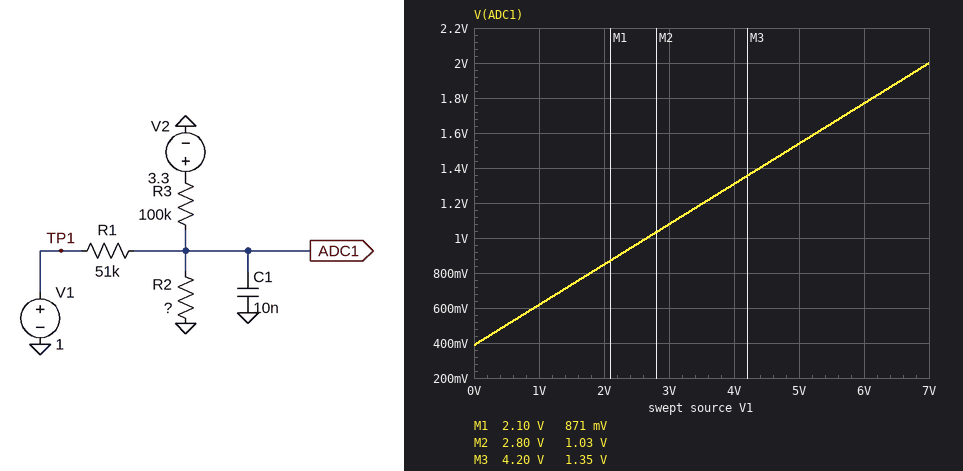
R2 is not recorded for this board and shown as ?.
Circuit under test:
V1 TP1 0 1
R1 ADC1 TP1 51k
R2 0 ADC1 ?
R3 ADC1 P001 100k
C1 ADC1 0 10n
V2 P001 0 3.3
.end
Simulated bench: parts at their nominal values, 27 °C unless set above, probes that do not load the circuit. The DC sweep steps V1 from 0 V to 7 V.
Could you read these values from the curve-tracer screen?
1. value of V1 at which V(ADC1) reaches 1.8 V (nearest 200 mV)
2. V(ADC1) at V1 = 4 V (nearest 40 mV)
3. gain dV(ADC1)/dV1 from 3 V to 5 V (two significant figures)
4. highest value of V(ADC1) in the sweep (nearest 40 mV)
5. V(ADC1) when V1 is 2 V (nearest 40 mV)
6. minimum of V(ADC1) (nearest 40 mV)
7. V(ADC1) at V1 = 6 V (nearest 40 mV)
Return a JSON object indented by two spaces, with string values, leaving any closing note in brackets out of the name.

{
  "value of V1 at which V(ADC1) reaches 1.8 V": "6.2 V",
  "V(ADC1) at V1 = 4 V": "1.32 V",
  "gain dV(ADC1)/dV1 from 3 V to 5 V": "0.23 V/V",
  "highest value of V(ADC1) in the sweep": "2.00 V",
  "V(ADC1) when V1 is 2 V": "840 mV",
  "minimum of V(ADC1)": "400 mV",
  "V(ADC1) at V1 = 6 V": "1.76 V"
}
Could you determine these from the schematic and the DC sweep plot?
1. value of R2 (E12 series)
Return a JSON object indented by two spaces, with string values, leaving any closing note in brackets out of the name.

{
  "value of R2": "18 kΩ"
}
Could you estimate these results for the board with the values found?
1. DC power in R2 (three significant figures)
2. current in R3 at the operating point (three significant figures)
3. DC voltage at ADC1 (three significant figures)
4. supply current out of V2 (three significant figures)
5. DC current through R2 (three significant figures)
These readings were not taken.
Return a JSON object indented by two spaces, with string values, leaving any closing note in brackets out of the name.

{
  "DC power in R2": "21.2 µW",
  "current in R3 at the operating point": "26.8 µA",
  "DC voltage at ADC1": "618 mV",
  "supply current out of V2": "26.8 µA",
  "DC current through R2": "34.3 µA"
}
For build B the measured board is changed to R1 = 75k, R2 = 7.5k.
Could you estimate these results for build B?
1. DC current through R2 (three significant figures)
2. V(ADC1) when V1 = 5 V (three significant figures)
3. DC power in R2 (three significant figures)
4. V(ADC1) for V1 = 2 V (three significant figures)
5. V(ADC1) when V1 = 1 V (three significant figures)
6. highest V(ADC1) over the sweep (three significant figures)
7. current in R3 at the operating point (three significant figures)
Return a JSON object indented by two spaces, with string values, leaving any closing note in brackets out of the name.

{
  "DC current through R2": "39.4 µA",
  "V(ADC1) when V1 = 5 V": "636 mV",
  "DC power in R2": "11.7 µW",
  "V(ADC1) for V1 = 2 V": "381 mV",
  "V(ADC1) when V1 = 1 V": "296 mV",
  "highest V(ADC1) over the sweep": "806 mV",
  "current in R3 at the operating point": "30.0 µA"
}
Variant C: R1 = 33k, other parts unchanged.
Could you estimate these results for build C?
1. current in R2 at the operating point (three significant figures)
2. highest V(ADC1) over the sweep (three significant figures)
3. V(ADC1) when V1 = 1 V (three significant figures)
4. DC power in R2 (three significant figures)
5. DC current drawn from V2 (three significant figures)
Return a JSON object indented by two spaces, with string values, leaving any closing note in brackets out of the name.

{
  "current in R2 at the operating point": "36.7 µA",
  "highest V(ADC1) over the sweep": "2.56 V",
  "V(ADC1) when V1 = 1 V": "660 mV",
  "DC power in R2": "24.2 µW",
  "DC current drawn from V2": "26.4 µA"
}
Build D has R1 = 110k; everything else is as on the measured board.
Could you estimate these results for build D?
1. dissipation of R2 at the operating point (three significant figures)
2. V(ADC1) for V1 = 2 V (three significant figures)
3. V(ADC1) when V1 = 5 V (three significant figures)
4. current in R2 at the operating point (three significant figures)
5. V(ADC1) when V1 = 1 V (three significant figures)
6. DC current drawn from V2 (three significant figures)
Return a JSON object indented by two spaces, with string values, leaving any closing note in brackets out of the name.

{
  "dissipation of R2 at the operating point": "17.7 µW",
  "V(ADC1) for V1 = 2 V": "686 mV",
  "V(ADC1) when V1 = 5 V": "1.05 V",
  "current in R2 at the operating point": "31.3 µA",
  "V(ADC1) when V1 = 1 V": "564 mV",
  "DC current drawn from V2": "27.4 µA"
}
